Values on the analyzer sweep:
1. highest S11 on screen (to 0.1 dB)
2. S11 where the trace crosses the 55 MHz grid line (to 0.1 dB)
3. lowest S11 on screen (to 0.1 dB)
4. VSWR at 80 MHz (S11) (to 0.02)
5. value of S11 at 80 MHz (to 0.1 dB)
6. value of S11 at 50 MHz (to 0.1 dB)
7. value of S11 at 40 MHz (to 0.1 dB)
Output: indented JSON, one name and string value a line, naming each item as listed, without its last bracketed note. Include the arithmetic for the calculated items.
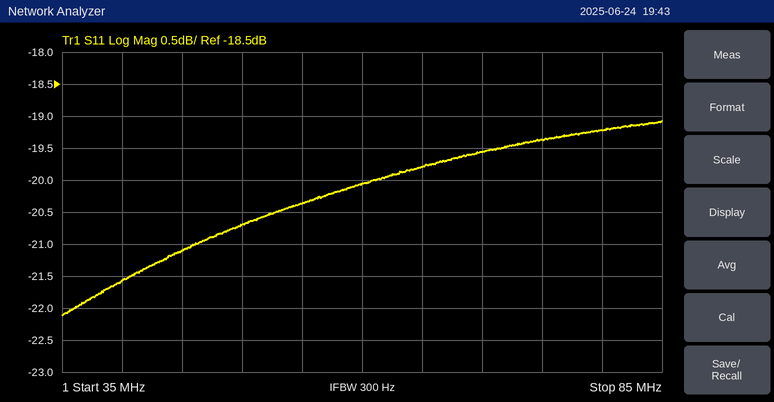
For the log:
{
  "highest S11 on screen": "-19.1 dB",
  "S11 where the trace crosses the 55 MHz grid line": "-20.4 dB",
  "lowest S11 on screen": "-22.1 dB",
  "VSWR at 80 MHz (S11)": "|Γ| = 10^(-19.2/20) = 0.1096; VSWR = (1 + 0.1096)/(1 − 0.1096) ≈ 1.25, so 1.24 to the nearest 0.02",
  "value of S11 at 80 MHz": "-19.2 dB",
  "value of S11 at 50 MHz": "-20.7 dB",
  "value of S11 at 40 MHz": "-21.6 dB"
}
